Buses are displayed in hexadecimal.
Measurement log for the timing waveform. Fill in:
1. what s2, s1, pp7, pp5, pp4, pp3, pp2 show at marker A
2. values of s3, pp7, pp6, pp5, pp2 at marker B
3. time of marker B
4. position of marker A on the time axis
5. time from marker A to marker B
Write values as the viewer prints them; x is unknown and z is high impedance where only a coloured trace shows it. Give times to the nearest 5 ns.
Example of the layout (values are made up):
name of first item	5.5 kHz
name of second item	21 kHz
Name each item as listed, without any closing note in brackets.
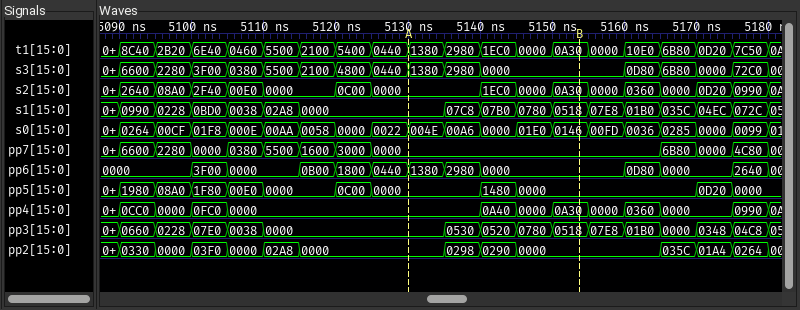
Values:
what s2, s1, pp7, pp5, pp4, pp3, pp2 show at marker A	s2=0000, s1=0000, pp7=0000, pp5=0000, pp4=0000, pp3=0000, pp2=0000
values of s3, pp7, pp6, pp5, pp2 at marker B	s3=0000, pp7=0000, pp6=0000, pp5=0000, pp2=0000
time of marker B	5155 ns
position of marker A on the time axis	5130 ns
time from marker A to marker B	25 ns
